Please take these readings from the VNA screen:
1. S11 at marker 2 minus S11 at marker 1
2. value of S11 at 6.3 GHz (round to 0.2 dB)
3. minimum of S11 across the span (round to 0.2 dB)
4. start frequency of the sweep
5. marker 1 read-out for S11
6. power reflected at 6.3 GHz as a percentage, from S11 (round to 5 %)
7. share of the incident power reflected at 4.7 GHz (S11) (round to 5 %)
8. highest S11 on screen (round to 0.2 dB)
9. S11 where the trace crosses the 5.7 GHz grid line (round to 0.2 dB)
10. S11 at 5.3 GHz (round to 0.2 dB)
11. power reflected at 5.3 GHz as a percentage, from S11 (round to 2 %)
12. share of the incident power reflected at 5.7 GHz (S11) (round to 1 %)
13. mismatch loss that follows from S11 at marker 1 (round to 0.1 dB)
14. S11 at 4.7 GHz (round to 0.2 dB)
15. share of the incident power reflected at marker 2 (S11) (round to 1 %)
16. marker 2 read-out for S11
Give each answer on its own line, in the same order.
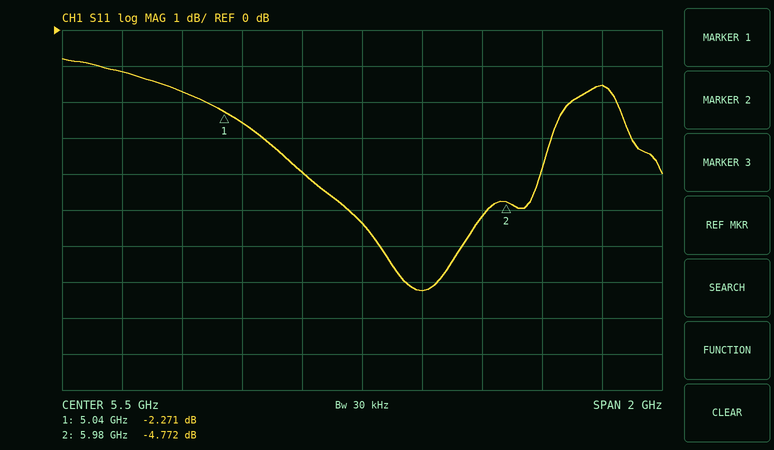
-2.501 dB
-1.6 dB
-7.2 dB
4.5 GHz
-2.271 dB
70 %
75 %
-0.8 dB
-7.2 dB
-4.0 dB
40 %
19 %
3.9 dB
-1.2 dB
33 %
-4.772 dB
